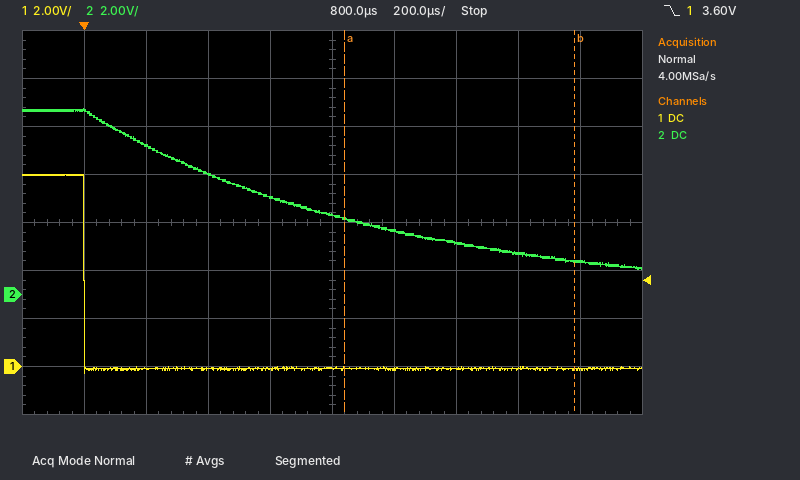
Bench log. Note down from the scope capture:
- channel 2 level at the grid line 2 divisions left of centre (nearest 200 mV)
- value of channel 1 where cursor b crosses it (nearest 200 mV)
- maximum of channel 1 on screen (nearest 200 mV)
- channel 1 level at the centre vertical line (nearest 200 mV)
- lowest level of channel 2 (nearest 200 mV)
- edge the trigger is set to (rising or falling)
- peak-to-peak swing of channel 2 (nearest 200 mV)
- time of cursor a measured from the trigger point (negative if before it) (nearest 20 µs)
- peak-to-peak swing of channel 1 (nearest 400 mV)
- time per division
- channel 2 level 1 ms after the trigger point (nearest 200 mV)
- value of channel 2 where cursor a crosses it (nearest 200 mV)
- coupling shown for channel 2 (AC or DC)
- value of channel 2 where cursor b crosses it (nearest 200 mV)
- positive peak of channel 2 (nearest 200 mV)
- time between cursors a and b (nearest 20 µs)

5.0 V
-200 mV
8.0 V
0.0 V
1.0 V
falling
6.8 V
+840 µs
8.4 V
200 µs
2.6 V
3.2 V
DC
1.4 V
7.8 V
740 µs
